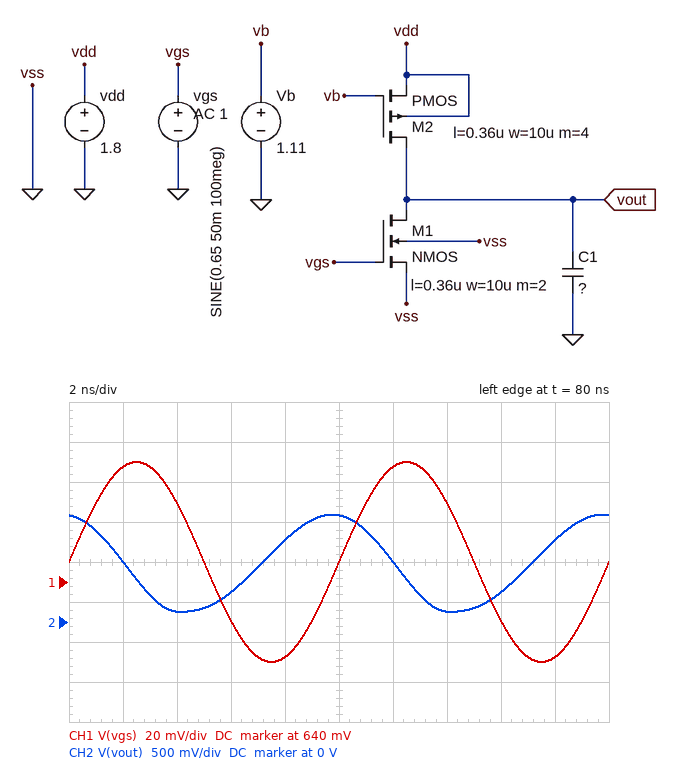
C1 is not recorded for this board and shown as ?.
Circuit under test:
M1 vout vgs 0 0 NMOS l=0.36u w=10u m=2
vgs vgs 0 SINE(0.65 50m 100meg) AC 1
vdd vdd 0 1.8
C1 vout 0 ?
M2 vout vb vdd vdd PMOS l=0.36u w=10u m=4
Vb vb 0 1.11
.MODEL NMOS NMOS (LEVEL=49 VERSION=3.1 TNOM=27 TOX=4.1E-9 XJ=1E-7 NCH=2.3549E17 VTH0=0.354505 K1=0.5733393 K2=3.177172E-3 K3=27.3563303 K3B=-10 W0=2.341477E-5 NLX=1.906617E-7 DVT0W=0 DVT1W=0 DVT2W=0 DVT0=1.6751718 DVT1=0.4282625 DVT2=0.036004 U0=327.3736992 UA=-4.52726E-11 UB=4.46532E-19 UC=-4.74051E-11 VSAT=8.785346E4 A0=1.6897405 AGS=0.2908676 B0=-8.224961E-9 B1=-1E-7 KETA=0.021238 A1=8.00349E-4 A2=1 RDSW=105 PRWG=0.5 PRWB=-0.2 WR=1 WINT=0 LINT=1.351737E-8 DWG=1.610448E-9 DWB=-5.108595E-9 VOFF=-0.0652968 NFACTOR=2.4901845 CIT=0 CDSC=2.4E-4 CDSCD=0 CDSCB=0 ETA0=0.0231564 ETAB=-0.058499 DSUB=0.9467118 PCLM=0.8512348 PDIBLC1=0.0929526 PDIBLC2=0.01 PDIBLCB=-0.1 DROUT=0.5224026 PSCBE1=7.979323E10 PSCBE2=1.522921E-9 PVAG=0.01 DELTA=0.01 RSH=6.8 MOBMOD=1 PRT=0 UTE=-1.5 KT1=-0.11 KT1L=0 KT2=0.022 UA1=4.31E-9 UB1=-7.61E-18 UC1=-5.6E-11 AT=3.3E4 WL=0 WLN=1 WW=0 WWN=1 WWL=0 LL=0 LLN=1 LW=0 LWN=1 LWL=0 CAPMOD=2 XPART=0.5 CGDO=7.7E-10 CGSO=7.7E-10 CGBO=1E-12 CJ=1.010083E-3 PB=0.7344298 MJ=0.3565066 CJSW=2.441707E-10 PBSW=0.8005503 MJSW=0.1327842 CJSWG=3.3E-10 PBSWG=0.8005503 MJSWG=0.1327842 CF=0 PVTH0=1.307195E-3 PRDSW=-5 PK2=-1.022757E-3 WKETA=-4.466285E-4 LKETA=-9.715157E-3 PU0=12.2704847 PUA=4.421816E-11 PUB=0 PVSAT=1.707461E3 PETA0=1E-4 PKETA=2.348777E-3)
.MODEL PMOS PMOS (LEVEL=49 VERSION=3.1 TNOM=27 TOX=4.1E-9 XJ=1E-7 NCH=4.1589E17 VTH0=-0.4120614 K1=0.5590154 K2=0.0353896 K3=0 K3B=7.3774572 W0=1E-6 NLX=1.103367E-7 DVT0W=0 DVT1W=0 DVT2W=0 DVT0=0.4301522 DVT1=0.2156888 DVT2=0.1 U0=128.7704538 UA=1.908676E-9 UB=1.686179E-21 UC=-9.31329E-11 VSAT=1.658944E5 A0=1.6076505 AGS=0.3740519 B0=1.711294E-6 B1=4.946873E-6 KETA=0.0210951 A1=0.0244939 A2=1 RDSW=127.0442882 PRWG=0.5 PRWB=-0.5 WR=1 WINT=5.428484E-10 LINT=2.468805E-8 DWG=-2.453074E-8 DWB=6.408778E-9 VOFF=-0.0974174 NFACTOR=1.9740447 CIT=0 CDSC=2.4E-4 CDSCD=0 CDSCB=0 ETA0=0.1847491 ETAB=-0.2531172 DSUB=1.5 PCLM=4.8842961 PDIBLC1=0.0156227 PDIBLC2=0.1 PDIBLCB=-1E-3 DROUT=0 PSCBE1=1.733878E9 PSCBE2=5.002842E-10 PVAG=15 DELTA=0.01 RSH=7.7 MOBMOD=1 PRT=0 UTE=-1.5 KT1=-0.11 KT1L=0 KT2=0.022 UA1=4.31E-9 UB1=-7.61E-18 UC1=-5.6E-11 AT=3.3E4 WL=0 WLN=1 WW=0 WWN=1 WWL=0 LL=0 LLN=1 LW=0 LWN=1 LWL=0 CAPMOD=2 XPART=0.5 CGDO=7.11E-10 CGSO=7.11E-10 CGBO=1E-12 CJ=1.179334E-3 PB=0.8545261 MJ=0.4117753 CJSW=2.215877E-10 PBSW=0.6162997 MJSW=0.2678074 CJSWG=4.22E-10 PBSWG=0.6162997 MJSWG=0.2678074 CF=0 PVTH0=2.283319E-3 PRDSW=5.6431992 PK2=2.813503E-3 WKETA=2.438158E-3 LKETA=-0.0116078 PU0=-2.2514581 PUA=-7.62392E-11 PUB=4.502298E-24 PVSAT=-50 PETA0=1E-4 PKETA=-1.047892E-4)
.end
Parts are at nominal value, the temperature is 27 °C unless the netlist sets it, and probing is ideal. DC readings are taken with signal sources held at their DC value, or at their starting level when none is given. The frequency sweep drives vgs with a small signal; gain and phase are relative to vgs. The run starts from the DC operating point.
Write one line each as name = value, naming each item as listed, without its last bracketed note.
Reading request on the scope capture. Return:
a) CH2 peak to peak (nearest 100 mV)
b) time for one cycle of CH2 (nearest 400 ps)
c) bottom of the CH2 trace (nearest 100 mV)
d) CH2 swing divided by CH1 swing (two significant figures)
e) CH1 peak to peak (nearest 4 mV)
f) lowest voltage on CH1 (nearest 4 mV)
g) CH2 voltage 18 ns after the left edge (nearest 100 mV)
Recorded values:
CH2 peak to peak = 1.2 V
time for one cycle of CH2 = 10.0 ns
bottom of the CH2 trace = 100 mV
CH2 swing divided by CH1 swing = 12
CH1 peak to peak = 100 mV
lowest voltage on CH1 = 600 mV
CH2 voltage 18 ns after the left edge = 1.0 V
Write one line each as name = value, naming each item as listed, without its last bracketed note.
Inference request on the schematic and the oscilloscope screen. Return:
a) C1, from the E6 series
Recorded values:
C1, from the E6 series = 220 fF
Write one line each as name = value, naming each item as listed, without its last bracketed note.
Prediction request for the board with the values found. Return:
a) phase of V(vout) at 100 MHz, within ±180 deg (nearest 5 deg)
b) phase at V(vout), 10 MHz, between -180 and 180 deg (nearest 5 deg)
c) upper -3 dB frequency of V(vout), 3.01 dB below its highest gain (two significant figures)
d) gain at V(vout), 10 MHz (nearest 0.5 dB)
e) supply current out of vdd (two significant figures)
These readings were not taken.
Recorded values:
phase of V(vout) at 100 MHz, within ±180 deg = 100 deg
phase at V(vout), 10 MHz, between -180 and 180 deg = 155 deg
upper -3 dB frequency of V(vout), 3.01 dB below its highest gain = 22 MHz
gain at V(vout), 10 MHz = 35.0 dB
supply current out of vdd = 190 µA
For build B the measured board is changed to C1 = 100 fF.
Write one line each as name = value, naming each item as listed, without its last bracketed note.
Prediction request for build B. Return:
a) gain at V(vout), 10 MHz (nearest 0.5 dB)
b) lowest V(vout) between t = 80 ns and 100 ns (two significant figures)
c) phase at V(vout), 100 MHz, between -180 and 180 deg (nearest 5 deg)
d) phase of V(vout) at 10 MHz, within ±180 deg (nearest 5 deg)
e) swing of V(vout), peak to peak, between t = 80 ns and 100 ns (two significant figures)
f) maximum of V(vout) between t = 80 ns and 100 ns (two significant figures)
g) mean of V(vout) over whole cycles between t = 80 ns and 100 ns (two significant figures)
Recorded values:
gain at V(vout), 10 MHz = 35.5 dB
lowest V(vout) between t = 80 ns and 100 ns = 93 mV
phase at V(vout), 100 MHz, between -180 and 180 deg = 110 deg
phase of V(vout) at 10 MHz, within ±180 deg = 165 deg
swing of V(vout), peak to peak, between t = 80 ns and 100 ns = 1.6 V
maximum of V(vout) between t = 80 ns and 100 ns = 1.7 V
mean of V(vout) over whole cycles between t = 80 ns and 100 ns = 850 mV
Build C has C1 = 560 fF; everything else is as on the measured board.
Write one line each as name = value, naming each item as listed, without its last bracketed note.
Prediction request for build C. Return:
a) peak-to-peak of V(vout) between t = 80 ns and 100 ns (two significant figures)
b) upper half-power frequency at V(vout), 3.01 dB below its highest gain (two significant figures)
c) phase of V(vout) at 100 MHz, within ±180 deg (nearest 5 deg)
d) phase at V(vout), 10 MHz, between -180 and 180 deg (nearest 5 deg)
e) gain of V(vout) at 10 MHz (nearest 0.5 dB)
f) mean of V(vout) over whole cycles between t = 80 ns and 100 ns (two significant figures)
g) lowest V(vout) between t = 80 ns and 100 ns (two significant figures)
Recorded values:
peak-to-peak of V(vout) between t = 80 ns and 100 ns = 580 mV
upper half-power frequency at V(vout), 3.01 dB below its highest gain = 9.8 MHz
phase of V(vout) at 100 MHz, within ±180 deg = 95 deg
phase at V(vout), 10 MHz, between -180 and 180 deg = 135 deg
gain of V(vout) at 10 MHz = 32.5 dB
mean of V(vout) over whole cycles between t = 80 ns and 100 ns = 600 mV
lowest V(vout) between t = 80 ns and 100 ns = 310 mV
